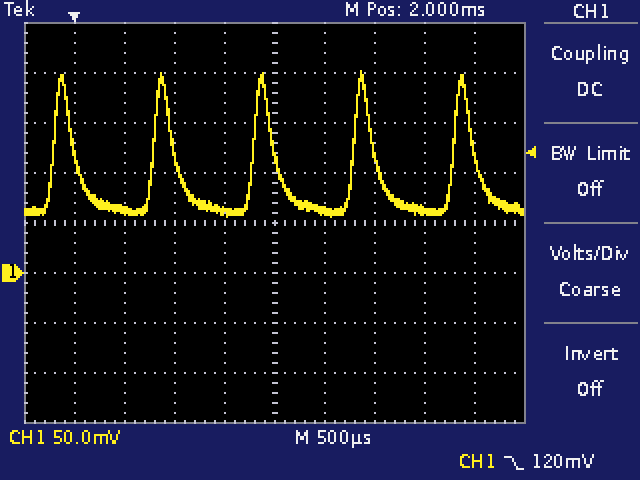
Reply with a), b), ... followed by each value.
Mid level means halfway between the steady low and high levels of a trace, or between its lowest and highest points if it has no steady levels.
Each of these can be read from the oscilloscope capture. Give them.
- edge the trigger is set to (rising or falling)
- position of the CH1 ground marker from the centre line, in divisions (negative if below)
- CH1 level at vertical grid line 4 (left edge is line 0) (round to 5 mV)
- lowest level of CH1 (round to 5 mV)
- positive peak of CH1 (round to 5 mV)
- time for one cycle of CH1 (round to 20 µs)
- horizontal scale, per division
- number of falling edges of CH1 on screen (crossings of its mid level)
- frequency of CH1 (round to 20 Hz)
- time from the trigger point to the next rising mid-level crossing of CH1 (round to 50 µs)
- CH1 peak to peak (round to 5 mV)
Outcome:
a) falling
b) -1.0 div
c) 60 mV
d) 55 mV
e) 200 mV
f) 1.00 ms
g) 500 µs
h) 5
i) 1.00 kHz
j) 800 µs
k) 145 mV
